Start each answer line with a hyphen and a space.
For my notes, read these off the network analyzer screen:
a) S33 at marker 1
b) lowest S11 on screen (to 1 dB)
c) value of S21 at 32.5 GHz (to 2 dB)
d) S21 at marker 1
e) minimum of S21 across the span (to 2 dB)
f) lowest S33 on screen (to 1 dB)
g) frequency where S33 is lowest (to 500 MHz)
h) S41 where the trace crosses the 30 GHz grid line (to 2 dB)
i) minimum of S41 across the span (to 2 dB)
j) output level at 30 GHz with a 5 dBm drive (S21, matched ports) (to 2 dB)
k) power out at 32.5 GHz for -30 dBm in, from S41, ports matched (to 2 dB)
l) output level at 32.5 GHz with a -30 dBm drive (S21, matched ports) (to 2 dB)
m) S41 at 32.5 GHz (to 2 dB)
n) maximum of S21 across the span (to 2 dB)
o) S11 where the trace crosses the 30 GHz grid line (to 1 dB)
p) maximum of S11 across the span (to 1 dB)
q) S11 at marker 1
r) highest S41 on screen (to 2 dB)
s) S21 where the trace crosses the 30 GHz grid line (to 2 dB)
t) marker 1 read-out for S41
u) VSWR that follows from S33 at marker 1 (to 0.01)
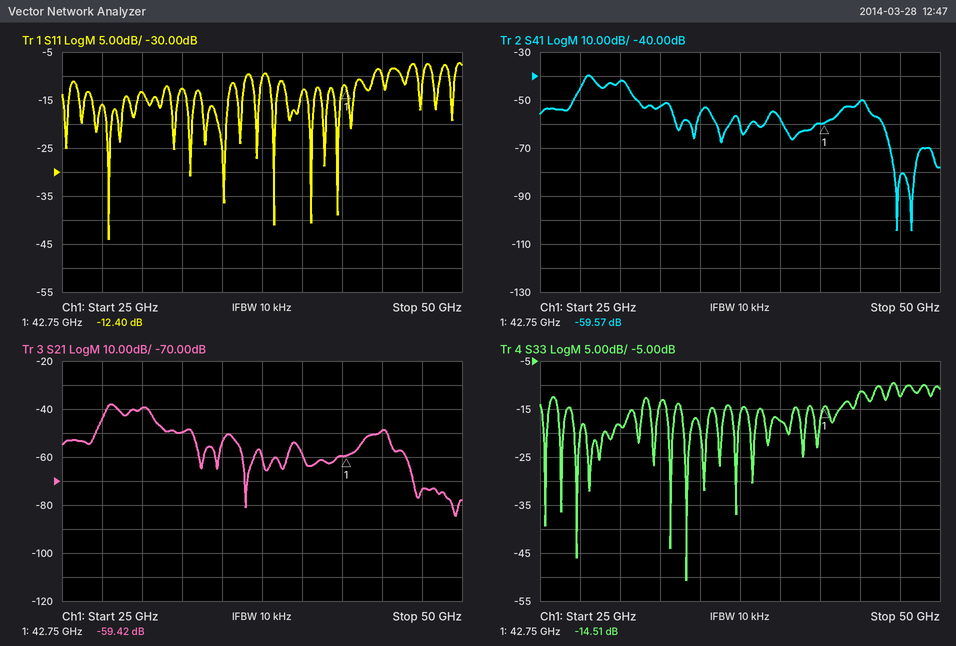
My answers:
- -14.51 dB
- -44 dB
- -50 dB
- -59.42 dB
- -84 dB
- -51 dB
- 34.0 GHz
- -42 dB
- -104 dB
- -34 dBm
- -82 dBm
- -80 dBm
- -52 dB
- -38 dB
- -13 dB
- -7 dB
- -12.40 dB
- -40 dB
- -40 dB
- -59.57 dB
- 1.46
